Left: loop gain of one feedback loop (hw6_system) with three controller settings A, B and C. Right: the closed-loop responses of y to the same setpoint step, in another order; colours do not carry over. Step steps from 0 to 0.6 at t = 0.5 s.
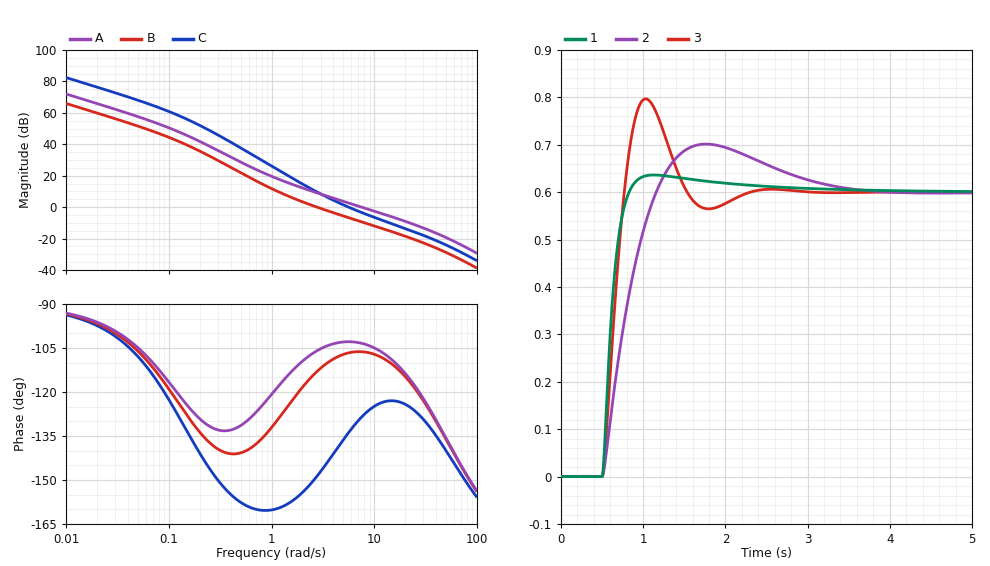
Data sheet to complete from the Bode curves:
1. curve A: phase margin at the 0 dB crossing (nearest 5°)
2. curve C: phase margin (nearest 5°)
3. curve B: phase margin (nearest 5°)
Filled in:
75°
45°
65°
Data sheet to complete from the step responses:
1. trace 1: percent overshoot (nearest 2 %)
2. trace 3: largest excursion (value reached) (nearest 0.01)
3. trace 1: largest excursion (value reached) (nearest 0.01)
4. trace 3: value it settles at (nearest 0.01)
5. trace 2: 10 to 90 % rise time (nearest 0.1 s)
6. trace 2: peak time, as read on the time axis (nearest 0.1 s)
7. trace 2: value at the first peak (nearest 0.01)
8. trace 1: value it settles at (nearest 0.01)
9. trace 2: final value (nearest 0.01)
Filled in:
6 %
0.80
0.64
0.60
0.5 s
1.8 s
0.70
0.60
0.60
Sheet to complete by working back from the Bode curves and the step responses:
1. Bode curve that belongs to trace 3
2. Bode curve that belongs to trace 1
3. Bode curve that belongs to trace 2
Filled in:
C
A
B
